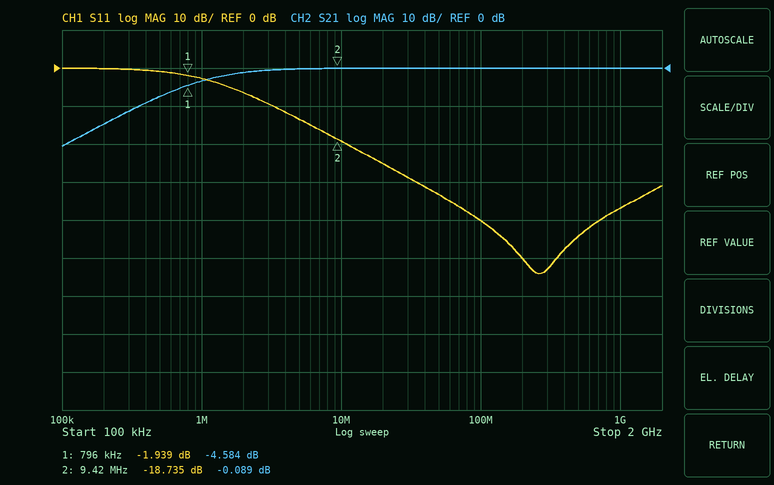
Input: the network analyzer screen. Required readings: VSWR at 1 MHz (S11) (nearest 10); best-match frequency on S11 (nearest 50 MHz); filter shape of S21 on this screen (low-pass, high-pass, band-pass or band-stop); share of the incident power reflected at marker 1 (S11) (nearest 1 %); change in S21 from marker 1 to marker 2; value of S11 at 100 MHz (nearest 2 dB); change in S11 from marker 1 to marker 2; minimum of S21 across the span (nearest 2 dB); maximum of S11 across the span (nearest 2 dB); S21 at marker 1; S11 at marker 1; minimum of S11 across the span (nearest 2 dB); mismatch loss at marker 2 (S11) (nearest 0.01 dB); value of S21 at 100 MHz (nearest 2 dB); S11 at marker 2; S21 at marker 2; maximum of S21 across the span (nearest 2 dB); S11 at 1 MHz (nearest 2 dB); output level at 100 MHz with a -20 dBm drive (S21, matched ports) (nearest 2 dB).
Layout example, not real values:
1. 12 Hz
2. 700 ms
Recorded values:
1. 10
2. 250 MHz
3. high-pass
4. 64 %
5. 4.495 dB
6. -40 dB
7. -16.796 dB
8. -20 dB
9. 0 dB
10. -4.584 dB
11. -1.939 dB
12. -54 dB
13. 0.06 dB
14. 0 dB
15. -18.735 dB
16. -0.089 dB
17. 0 dB
18. -2 dB
19. -20 dBm
